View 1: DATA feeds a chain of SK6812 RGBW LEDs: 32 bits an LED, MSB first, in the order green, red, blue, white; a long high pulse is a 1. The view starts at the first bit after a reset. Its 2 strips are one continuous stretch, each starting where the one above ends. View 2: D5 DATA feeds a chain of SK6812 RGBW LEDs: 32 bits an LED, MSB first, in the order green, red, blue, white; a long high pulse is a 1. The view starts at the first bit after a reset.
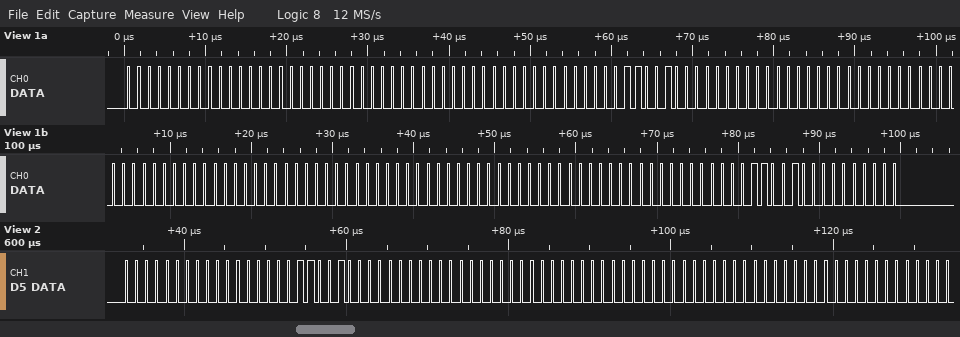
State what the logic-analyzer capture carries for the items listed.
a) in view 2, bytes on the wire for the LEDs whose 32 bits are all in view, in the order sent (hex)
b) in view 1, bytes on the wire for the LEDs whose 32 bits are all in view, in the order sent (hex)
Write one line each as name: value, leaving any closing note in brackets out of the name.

in view 2, bytes on the wire for the LEDs whose 32 bits are all in view, in the order sent: 00 00 64 00 00 00 00 00
in view 1, bytes on the wire for the LEDs whose 32 bits are all in view, in the order sent: 00 00 00 00 00 00 64 00 00 00 00 00 00 00 00 00 00 00 64 00
